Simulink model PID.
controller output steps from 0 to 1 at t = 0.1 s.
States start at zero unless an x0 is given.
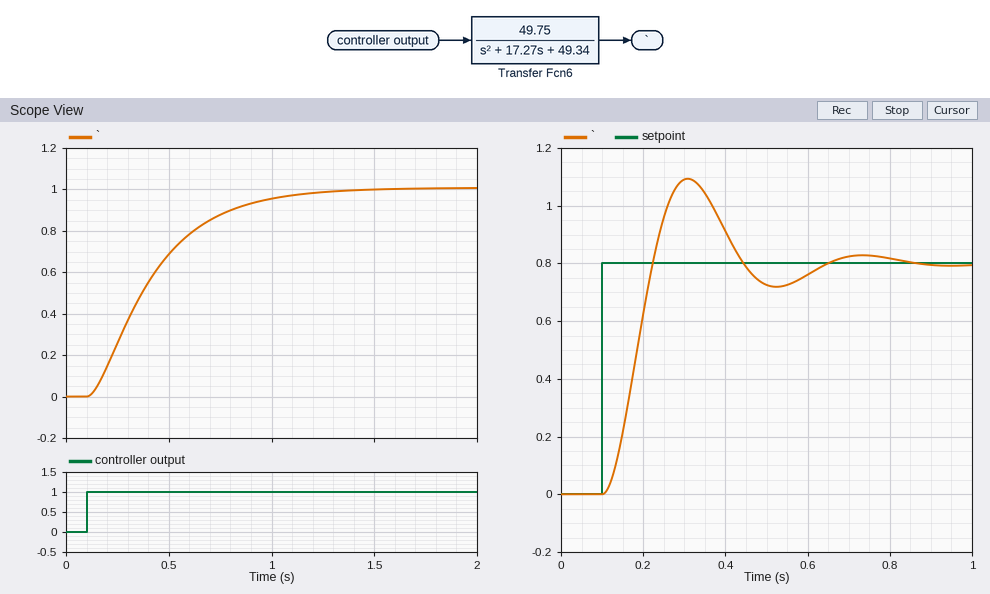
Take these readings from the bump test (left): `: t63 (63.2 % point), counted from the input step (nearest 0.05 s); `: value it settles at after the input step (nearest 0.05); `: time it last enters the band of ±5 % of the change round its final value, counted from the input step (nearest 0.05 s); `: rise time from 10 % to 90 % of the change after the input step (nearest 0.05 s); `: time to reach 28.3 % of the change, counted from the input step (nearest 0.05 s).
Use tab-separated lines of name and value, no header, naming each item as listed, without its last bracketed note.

`: t63 (63.2 % point), counted from the input step	0.35 s
`: value it settles at after the input step	1.00
`: time it last enters the band of ±5 % of the change round its final value, counted from the input step	0.90 s
`: rise time from 10 % to 90 % of the change after the input step	0.65 s
`: time to reach 28.3 % of the change, counted from the input step	0.15 s
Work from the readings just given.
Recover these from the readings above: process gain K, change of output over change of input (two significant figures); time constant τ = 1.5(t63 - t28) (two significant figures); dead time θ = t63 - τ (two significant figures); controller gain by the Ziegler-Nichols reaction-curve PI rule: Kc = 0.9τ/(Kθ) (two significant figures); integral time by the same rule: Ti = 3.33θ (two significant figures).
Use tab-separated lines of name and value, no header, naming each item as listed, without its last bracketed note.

process gain K, change of output over change of input	1.0
time constant τ = 1.5(t63 - t28)	0.30 s
dead time θ = t63 - τ	0.050 s
controller gain by the Ziegler-Nichols reaction-curve PI rule: Kc = 0.9τ/(Kθ)	5.4
integral time by the same rule: Ti = 3.33θ	0.17 s
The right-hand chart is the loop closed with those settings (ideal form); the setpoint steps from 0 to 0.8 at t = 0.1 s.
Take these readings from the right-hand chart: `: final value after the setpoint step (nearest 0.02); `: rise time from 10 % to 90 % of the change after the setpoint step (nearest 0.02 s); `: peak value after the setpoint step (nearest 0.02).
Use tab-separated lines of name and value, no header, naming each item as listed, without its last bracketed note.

`: final value after the setpoint step	0.80
`: rise time from 10 % to 90 % of the change after the setpoint step	0.08 s
`: peak value after the setpoint step	1.10
